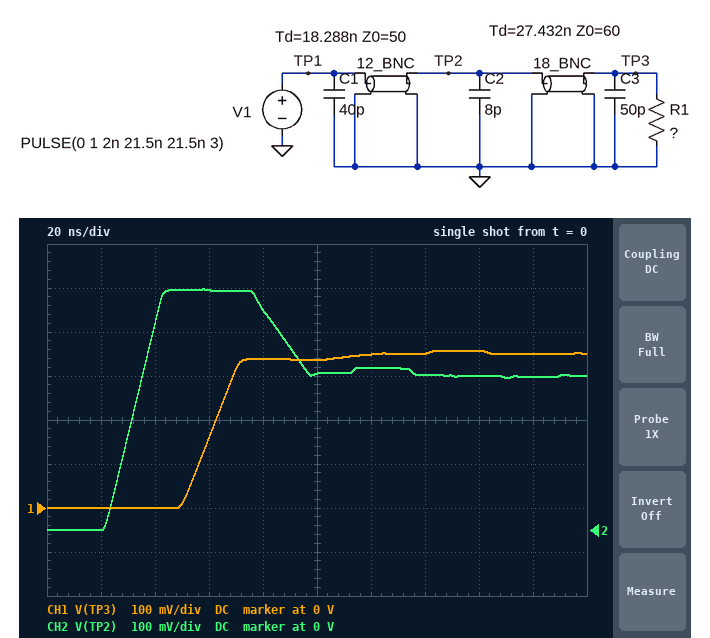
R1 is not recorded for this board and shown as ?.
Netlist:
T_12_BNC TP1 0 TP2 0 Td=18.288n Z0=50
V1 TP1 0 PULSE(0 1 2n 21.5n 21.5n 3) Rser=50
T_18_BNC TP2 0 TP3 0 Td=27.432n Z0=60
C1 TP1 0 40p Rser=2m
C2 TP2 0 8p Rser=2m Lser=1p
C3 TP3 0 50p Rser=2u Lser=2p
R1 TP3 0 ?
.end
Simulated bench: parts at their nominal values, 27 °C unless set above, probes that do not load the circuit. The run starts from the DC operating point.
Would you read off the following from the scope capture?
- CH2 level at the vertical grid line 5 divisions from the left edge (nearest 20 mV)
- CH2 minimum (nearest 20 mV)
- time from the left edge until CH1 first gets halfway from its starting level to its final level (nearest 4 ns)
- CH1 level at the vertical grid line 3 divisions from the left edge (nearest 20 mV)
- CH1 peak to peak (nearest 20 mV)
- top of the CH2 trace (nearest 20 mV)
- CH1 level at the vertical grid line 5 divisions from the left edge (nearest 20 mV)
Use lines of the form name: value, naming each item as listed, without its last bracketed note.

CH2 level at the vertical grid line 5 divisions from the left edge: 360 mV
CH2 minimum: 0 V
time from the left edge until CH1 first gets halfway from its starting level to its final level: 60 ns
CH1 level at the vertical grid line 3 divisions from the left edge: 160 mV
CH1 peak to peak: 360 mV
top of the CH2 trace: 540 mV
CH1 level at the vertical grid line 5 divisions from the left edge: 340 mV
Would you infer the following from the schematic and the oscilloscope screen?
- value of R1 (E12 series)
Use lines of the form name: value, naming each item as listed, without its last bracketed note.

value of R1: 27 Ω
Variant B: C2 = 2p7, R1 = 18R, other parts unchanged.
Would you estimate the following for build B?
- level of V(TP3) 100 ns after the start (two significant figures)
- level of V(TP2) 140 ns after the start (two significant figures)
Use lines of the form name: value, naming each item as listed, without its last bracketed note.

level of V(TP3) 100 ns after the start: 250 mV
level of V(TP2) 140 ns after the start: 270 mV
